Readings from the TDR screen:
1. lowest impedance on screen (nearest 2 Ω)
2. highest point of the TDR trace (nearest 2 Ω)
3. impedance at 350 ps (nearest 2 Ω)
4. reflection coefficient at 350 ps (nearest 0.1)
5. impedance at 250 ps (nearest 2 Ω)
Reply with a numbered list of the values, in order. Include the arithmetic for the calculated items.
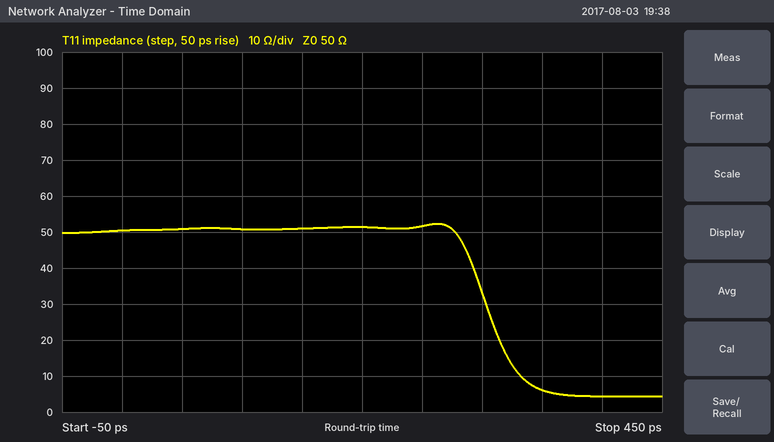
1. 4 Ω
2. 52 Ω
3. 6 Ω
4. (6 − 50)/(6 + 50) ≈ -0.8
5. 52 Ω
